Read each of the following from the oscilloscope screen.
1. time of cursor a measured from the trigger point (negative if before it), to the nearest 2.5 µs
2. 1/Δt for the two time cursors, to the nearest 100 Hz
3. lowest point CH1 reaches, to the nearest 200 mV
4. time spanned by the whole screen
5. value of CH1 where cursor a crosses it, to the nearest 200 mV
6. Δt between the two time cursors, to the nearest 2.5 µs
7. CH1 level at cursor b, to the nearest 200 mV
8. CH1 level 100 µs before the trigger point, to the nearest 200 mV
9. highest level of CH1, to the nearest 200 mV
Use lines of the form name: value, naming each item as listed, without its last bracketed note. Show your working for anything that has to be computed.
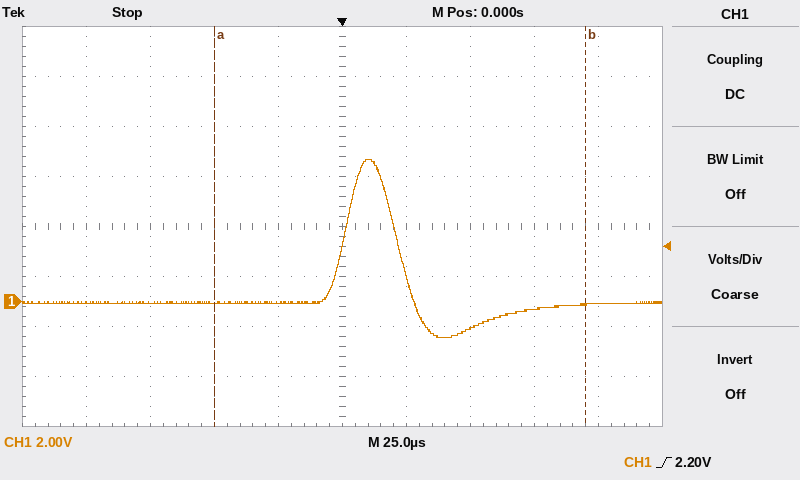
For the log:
time of cursor a measured from the trigger point (negative if before it), to the nearest 2.5 µs: -50.0 µs
1/Δt for the two time cursors, to the nearest 100 Hz: 1 / 145.0 µs ≈ 6.9 kHz
lowest point CH1 reaches, to the nearest 200 mV: -1.4 V
time spanned by the whole screen: 250 µs
value of CH1 where cursor a crosses it, to the nearest 200 mV: 0.0 V
Δt between the two time cursors, to the nearest 2.5 µs: 145.0 µs
CH1 level at cursor b, to the nearest 200 mV: -200 mV
CH1 level 100 µs before the trigger point, to the nearest 200 mV: 0.0 V
highest level of CH1, to the nearest 200 mV: 5.6 V
